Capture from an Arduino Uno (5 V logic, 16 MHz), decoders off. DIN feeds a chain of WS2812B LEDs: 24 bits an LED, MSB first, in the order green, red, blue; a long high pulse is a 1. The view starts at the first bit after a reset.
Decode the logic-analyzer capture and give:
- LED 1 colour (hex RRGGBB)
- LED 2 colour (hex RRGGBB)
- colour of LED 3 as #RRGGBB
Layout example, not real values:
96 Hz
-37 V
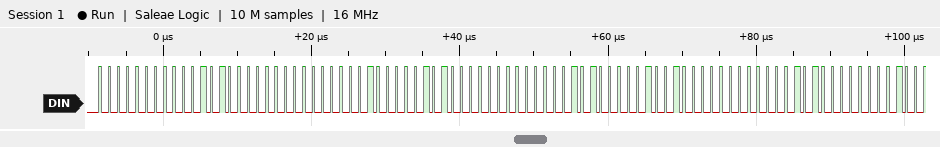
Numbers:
#140000
#140400
#121400
